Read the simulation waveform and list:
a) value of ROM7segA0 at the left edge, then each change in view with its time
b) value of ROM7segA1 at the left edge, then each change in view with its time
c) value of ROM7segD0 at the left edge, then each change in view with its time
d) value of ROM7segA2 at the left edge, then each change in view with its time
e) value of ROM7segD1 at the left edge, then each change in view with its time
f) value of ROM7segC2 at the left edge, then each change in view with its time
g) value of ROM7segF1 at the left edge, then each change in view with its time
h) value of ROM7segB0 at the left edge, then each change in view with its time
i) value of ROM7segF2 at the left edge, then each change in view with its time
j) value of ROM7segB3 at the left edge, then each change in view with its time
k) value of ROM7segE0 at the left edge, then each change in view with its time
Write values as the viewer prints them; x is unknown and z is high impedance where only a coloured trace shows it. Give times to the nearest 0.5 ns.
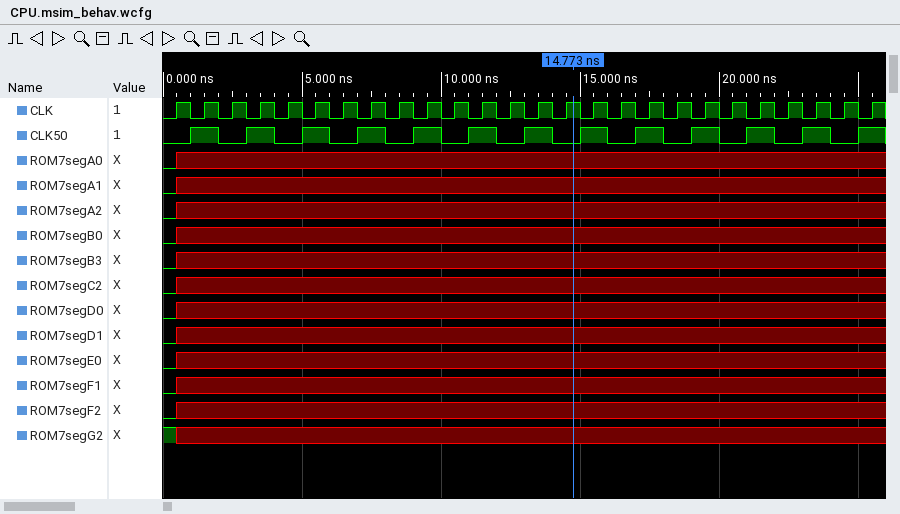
0, x at 0.5 ns
0, x at 0.5 ns
0, x at 0.5 ns
0, x at 0.5 ns
0, x at 0.5 ns
0, x at 0.5 ns
0, x at 0.5 ns
0, x at 0.5 ns
0, x at 0.5 ns
0, x at 0.5 ns
0, x at 0.5 ns
